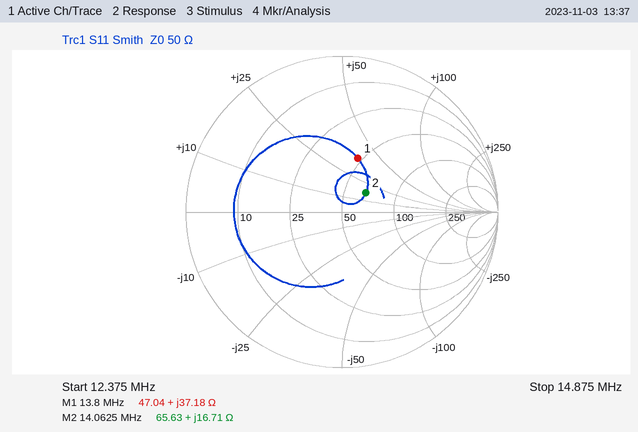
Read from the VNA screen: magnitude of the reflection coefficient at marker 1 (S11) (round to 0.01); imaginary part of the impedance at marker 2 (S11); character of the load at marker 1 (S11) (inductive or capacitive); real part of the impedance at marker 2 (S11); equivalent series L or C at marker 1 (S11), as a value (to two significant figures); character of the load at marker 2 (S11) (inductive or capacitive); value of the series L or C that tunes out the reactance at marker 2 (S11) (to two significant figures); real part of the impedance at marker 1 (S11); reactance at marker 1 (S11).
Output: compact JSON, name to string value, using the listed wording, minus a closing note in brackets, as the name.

{"magnitude of the reflection coefficient at marker 1 (S11)": "0.36", "imaginary part of the impedance at marker 2": "+16.71 Ω", "character of the load at marker 1 (S11)": "inductive", "real part of the impedance at marker 2": "65.63 Ω", "equivalent series L or C at marker 1 (S11), as a value": "430 nH", "character of the load at marker 2 (S11)": "inductive", "value of the series L or C that tunes out the reactance at marker 2 (S11)": "680 pF", "real part of the impedance at marker 1": "47.04 Ω", "reactance at marker 1": "+37.18 Ω"}
